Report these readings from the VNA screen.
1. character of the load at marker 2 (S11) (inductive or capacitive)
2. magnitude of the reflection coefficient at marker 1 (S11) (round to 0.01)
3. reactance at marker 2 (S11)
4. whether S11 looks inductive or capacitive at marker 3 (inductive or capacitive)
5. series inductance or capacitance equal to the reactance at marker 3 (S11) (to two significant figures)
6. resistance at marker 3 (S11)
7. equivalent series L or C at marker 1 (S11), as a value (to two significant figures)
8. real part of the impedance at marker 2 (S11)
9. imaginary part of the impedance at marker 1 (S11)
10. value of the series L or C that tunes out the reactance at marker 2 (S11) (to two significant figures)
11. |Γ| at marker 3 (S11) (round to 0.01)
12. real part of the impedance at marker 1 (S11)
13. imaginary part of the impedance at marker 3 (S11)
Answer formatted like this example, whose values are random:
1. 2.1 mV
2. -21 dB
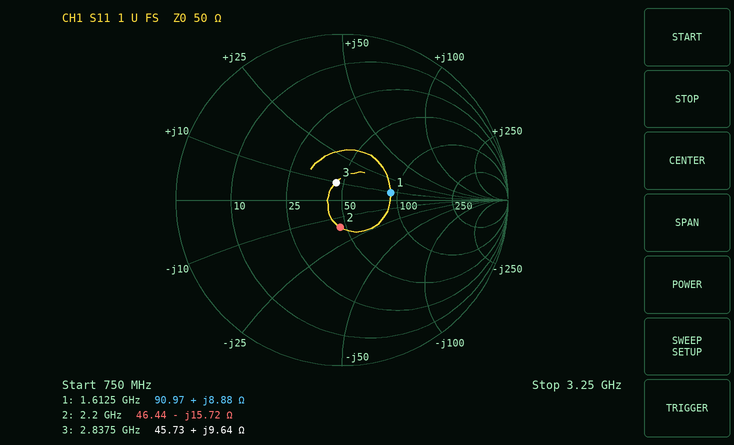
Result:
1. capacitive
2. 0.30
3. -15.72 Ω
4. inductive
5. 540 pH
6. 45.73 Ω
7. 880 pH
8. 46.44 Ω
9. +8.88 Ω
10. 1.1 nH
11. 0.11
12. 90.97 Ω
13. +9.64 Ω
